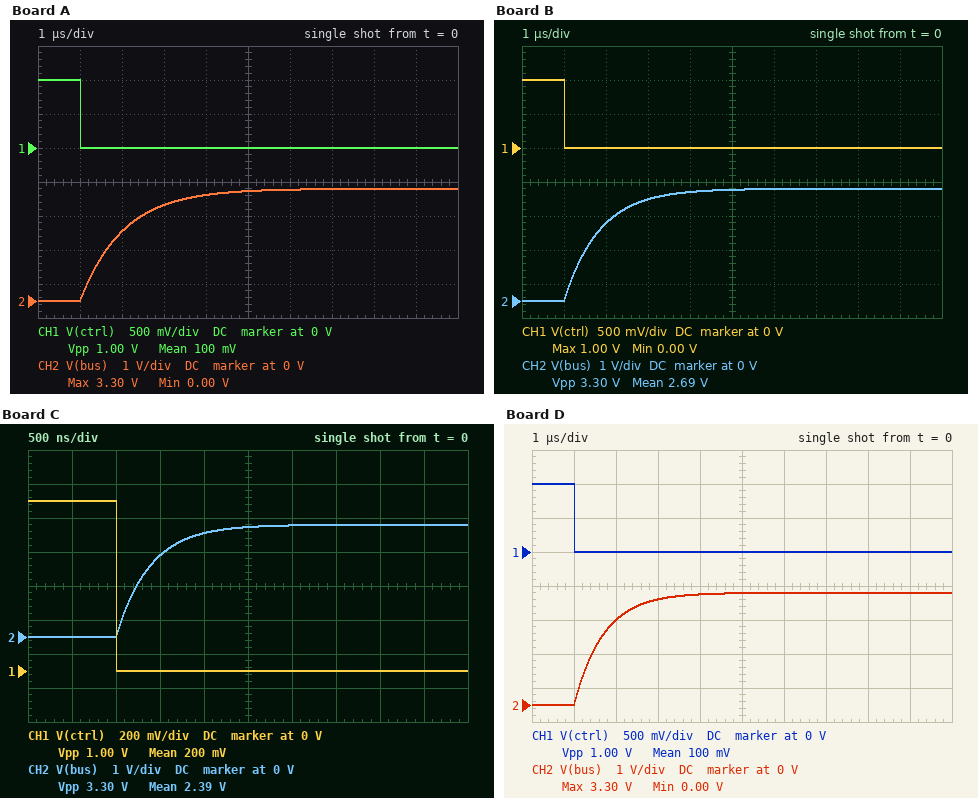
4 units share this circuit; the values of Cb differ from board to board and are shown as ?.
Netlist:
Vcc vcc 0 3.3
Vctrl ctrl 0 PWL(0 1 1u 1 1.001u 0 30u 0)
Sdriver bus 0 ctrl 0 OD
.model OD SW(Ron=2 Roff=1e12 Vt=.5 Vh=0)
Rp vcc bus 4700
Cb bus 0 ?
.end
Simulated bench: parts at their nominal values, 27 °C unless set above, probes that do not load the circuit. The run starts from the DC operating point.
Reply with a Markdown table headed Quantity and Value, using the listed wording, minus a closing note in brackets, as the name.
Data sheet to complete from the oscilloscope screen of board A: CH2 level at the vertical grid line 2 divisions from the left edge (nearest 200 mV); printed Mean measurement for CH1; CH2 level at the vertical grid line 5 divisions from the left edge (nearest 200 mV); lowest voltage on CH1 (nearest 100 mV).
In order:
| Quantity | Value |
|---|---|
| CH2 level at the vertical grid line 2 divisions from the left edge | 2.0 V |
| printed Mean measurement for CH1 | 100 mV |
| CH2 level at the vertical grid line 5 divisions from the left edge | 3.2 V |
| lowest voltage on CH1 | 0 V |
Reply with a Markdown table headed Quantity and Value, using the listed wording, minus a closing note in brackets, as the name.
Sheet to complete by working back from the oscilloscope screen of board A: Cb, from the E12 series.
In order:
| Quantity | Value |
|---|---|
| Cb, from the E12 series | 220 pF |
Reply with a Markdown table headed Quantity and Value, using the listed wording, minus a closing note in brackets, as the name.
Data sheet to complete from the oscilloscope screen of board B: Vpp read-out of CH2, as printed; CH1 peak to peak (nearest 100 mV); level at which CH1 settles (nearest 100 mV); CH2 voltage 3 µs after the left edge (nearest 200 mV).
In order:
| Quantity | Value |
|---|---|
| Vpp read-out of CH2, as printed | 3.30 V |
| CH1 peak to peak | 1.0 V |
| level at which CH1 settles | 0 V |
| CH2 voltage 3 µs after the left edge | 3.0 V |
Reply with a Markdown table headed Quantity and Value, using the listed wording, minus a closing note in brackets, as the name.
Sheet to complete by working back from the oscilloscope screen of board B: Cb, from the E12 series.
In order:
| Quantity | Value |
|---|---|
| Cb, from the E12 series | 180 pF |
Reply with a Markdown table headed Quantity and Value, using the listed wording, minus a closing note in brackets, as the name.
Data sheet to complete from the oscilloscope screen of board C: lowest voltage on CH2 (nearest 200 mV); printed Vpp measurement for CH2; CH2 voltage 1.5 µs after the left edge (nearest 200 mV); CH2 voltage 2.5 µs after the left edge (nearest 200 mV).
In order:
| Quantity | Value |
|---|---|
| lowest voltage on CH2 | 0 V |
| printed Vpp measurement for CH2 | 3.30 V |
| CH2 voltage 1.5 µs after the left edge | 2.4 V |
| CH2 voltage 2.5 µs after the left edge | 3.2 V |
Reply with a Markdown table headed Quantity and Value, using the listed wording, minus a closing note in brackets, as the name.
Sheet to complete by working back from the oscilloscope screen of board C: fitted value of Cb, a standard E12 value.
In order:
| Quantity | Value |
|---|---|
| fitted value of Cb, a standard E12 value | 82 pF |
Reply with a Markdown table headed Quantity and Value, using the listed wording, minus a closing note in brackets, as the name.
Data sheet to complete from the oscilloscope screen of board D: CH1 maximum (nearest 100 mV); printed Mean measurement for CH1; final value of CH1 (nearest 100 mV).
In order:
| Quantity | Value |
|---|---|
| CH1 maximum | 1.0 V |
| printed Mean measurement for CH1 | 100 mV |
| final value of CH1 | 0 V |
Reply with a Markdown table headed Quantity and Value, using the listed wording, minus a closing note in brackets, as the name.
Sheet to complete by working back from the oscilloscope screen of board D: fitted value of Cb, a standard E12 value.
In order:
| Quantity | Value |
|---|---|
| fitted value of Cb, a standard E12 value | 150 pF |
